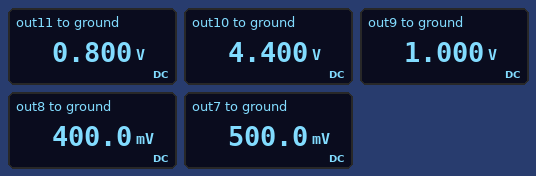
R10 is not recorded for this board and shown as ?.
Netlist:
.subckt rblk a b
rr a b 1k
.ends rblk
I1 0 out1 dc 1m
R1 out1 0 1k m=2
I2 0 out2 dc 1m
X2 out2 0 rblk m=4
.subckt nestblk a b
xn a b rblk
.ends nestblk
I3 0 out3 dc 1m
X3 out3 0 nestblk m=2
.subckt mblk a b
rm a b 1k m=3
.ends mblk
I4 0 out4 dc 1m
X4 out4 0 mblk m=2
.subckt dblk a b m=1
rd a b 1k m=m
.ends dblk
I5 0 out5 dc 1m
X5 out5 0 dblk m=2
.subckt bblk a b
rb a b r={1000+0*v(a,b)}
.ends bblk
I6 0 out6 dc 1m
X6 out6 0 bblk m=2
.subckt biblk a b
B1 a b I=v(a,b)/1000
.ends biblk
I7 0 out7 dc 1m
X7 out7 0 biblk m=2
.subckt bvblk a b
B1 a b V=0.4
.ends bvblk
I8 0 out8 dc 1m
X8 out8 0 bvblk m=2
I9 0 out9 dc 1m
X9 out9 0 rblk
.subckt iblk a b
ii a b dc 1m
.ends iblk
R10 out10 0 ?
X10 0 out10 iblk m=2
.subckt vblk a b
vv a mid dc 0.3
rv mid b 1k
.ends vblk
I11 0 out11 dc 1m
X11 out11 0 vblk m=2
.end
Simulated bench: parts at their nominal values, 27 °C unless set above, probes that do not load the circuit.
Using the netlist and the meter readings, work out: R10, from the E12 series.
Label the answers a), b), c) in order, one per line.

a) 2.2 kΩ
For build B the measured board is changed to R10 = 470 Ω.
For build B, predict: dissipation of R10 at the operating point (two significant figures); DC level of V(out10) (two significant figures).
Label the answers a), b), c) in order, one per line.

a) 1.9 mW
b) 940 mV
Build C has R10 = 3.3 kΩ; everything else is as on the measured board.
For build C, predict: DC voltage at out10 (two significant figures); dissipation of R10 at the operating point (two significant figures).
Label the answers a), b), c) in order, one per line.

a) 6.6 V
b) 13 mW
